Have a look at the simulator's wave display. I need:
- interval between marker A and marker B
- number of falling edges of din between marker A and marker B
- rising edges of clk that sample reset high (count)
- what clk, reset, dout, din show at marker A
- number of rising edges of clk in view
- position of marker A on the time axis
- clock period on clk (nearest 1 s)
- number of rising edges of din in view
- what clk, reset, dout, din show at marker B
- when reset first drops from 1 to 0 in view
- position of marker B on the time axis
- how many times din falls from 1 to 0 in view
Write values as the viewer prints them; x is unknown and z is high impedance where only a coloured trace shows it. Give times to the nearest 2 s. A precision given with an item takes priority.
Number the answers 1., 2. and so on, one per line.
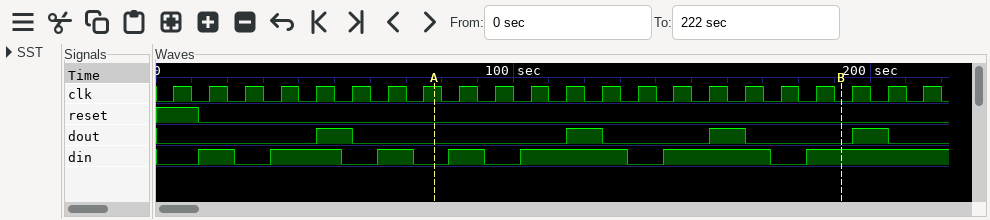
1. 114 s
2. 3
3. 1
4. clk=1, reset=0, dout=0, din=0
5. 22
6. 78 s
7. 10 s
8. 7
9. clk=0, reset=0, dout=0, din=1
10. 12 s
11. 192 s
12. 6
